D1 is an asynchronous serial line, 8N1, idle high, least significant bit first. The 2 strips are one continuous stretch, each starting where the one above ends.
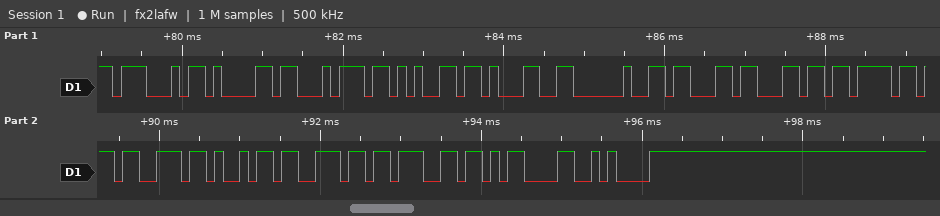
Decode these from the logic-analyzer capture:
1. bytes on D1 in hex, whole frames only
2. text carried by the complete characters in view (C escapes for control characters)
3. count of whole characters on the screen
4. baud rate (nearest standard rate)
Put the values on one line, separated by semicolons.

47 61 74 65 31 20 63 6C 6F 73 69 6E 67 0D 0A; "Gate1 closing\r\n"; 15; 9600 baud
